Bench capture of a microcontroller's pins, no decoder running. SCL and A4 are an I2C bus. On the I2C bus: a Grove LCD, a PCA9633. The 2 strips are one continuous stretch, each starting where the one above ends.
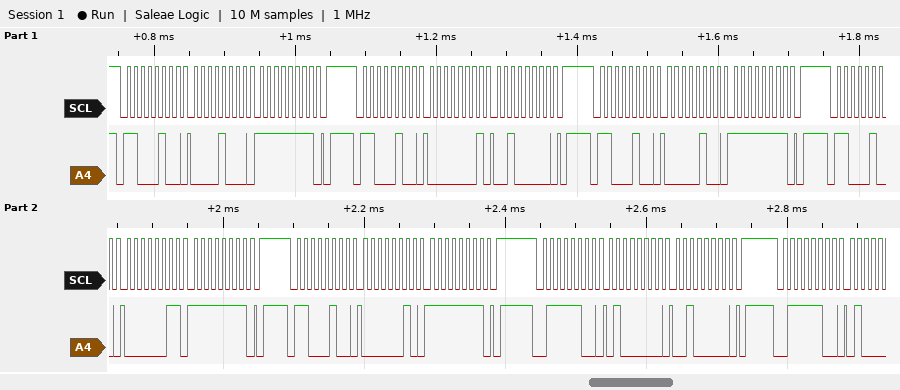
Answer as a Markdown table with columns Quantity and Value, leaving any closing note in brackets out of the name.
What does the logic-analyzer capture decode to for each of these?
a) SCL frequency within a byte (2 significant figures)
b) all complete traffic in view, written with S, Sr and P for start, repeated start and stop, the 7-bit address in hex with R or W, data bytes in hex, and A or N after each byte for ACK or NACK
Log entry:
| Quantity | Value |
|---|---|
| SCL frequency within a byte | 100 kHz |
| all complete traffic in view, written with S, Sr and P for start, repeated start and stop, the 7-bit address in hex with R or W, data bytes in hex, and A or N after each byte for ACK or NACK | S 62W A 08 A FF A P S 62W A 01 A 20 A P S 62W A 04 A FF A P S 62W A 03 A FF A P S 62W A 02 A FF A P S 3EW A 40 A 20 A P S 3EW A |
